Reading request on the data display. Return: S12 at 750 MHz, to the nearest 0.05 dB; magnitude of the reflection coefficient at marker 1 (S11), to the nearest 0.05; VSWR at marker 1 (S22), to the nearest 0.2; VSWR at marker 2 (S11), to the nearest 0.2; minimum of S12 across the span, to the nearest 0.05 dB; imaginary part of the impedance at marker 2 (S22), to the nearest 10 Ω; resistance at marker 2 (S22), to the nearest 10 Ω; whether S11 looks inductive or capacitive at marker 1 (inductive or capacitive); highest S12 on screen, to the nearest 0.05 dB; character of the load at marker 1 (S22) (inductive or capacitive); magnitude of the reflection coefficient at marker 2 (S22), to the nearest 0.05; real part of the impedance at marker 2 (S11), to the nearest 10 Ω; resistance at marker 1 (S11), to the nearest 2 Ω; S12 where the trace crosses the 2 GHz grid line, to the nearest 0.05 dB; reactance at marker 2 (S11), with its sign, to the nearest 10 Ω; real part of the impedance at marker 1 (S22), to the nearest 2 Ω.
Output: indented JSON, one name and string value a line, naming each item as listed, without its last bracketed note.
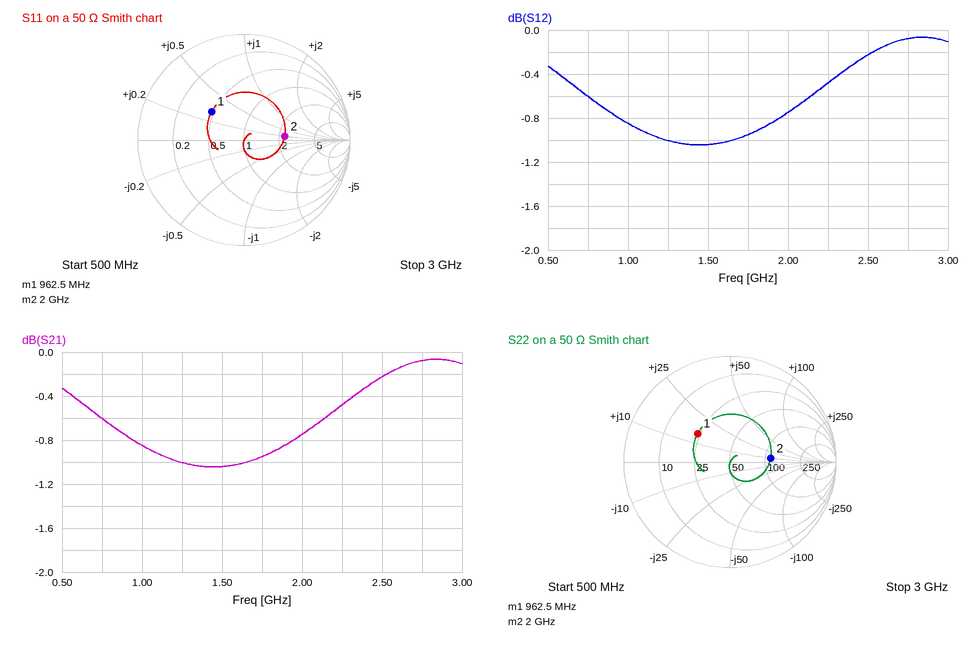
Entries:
{
  "S12 at 750 MHz, to the nearest 0.05 dB": "-0.60 dB",
  "magnitude of the reflection coefficient at marker 1 (S11), to the nearest 0.05": "0.40",
  "VSWR at marker 1 (S22), to the nearest 0.2": "2.4",
  "VSWR at marker 2 (S11), to the nearest 0.2": "2.2",
  "minimum of S12 across the span, to the nearest 0.05 dB": "-1.05 dB",
  "imaginary part of the impedance at marker 2 (S22), to the nearest 10 Ω": "+10 Ω",
  "resistance at marker 2 (S22), to the nearest 10 Ω": "110 Ω",
  "whether S11 looks inductive or capacitive at marker 1": "inductive",
  "highest S12 on screen, to the nearest 0.05 dB": "-0.05 dB",
  "character of the load at marker 1 (S22)": "inductive",
  "magnitude of the reflection coefficient at marker 2 (S22), to the nearest 0.05": "0.40",
  "real part of the impedance at marker 2 (S11), to the nearest 10 Ω": "110 Ω",
  "resistance at marker 1 (S11), to the nearest 2 Ω": "24 Ω",
  "S12 where the trace crosses the 2 GHz grid line, to the nearest 0.05 dB": "-0.75 dB",
  "reactance at marker 2 (S11), with its sign, to the nearest 10 Ω": "+10 Ω",
  "real part of the impedance at marker 1 (S22), to the nearest 2 Ω": "24 Ω"
}
